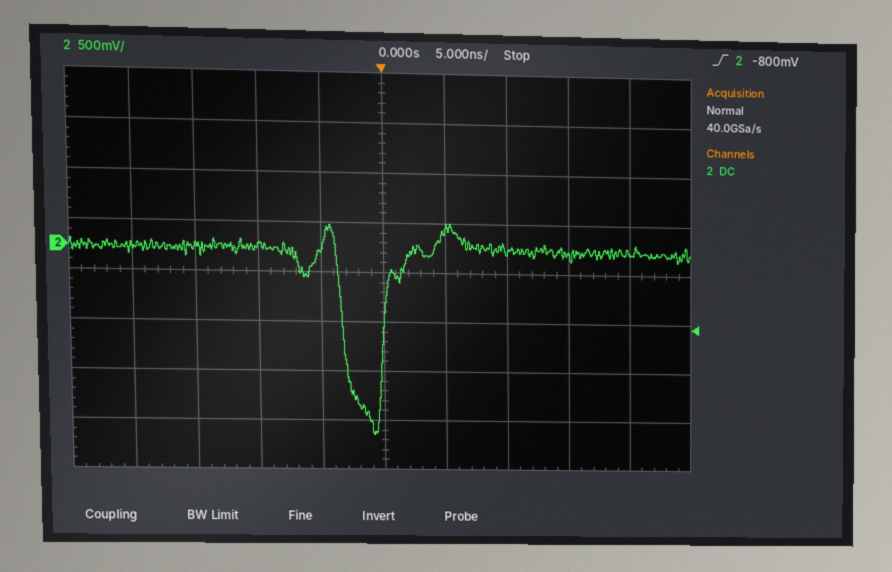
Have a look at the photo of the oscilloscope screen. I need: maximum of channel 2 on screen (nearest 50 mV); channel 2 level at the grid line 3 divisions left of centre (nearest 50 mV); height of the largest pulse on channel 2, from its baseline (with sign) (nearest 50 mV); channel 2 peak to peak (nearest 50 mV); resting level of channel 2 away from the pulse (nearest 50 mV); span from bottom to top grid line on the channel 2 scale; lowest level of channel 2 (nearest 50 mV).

250 mV
0 mV
-1.90 V
2.15 V
0 mV
4 V
-1.90 V
